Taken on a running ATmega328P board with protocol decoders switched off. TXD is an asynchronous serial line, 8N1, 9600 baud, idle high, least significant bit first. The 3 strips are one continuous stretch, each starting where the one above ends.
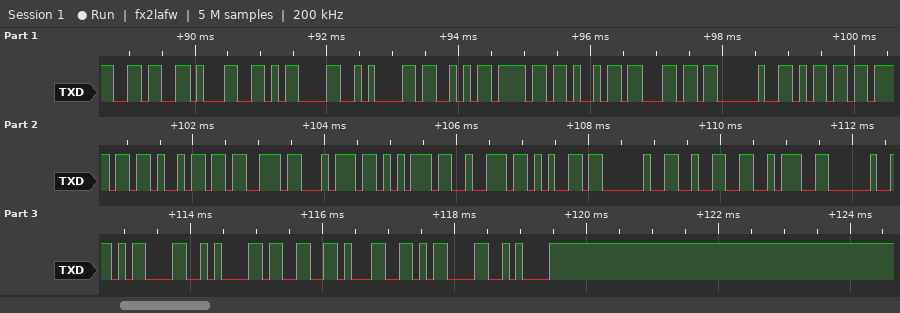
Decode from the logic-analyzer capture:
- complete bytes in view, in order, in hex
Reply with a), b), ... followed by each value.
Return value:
a) 0x36 0x31 0x0D 0x0A 0x53 0x6F 0x69 0x6C 0x20 0x6D 0x6F 0x69 0x73 0x74 0x75 0x72 0x65 0x20 0x32 0x3A 0x20 0x0D 0x0A 0x33 0x31 0x0D 0x0A
